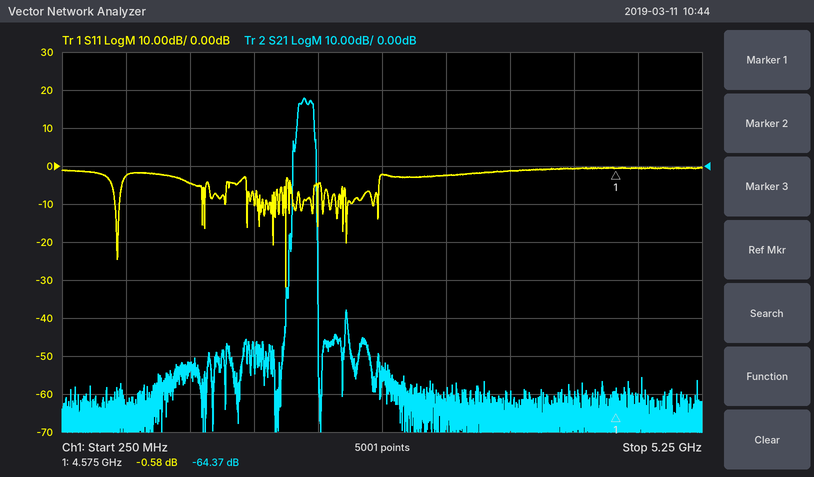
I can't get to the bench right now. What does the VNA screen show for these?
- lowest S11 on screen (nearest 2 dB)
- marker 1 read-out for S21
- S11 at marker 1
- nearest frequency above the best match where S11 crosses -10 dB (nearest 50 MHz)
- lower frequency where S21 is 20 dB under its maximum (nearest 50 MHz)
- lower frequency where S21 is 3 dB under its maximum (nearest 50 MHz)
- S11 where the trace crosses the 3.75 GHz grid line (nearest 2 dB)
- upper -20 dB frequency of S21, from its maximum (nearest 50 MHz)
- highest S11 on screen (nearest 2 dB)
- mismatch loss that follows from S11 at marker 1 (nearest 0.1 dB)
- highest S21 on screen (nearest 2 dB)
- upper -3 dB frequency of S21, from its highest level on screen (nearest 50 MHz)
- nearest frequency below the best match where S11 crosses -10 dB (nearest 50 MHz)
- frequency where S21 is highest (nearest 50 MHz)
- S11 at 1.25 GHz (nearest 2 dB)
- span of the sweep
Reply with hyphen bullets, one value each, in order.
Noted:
- -32 dB
- -64.37 dB
- -0.58 dB
- 2.00 GHz
- 2.05 GHz
- 2.10 GHz
- -2 dB
- 2.25 GHz
- 0 dB
- 9.0 dB
- 18 dB
- 2.20 GHz
- 2.00 GHz
- 2.15 GHz
- -4 dB
- 5 GHz
